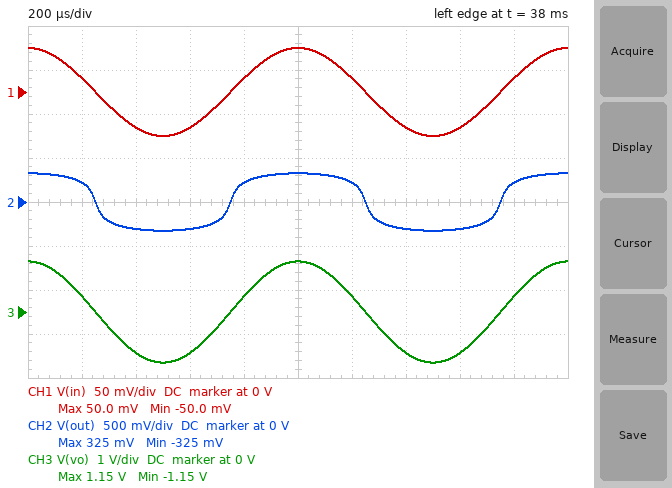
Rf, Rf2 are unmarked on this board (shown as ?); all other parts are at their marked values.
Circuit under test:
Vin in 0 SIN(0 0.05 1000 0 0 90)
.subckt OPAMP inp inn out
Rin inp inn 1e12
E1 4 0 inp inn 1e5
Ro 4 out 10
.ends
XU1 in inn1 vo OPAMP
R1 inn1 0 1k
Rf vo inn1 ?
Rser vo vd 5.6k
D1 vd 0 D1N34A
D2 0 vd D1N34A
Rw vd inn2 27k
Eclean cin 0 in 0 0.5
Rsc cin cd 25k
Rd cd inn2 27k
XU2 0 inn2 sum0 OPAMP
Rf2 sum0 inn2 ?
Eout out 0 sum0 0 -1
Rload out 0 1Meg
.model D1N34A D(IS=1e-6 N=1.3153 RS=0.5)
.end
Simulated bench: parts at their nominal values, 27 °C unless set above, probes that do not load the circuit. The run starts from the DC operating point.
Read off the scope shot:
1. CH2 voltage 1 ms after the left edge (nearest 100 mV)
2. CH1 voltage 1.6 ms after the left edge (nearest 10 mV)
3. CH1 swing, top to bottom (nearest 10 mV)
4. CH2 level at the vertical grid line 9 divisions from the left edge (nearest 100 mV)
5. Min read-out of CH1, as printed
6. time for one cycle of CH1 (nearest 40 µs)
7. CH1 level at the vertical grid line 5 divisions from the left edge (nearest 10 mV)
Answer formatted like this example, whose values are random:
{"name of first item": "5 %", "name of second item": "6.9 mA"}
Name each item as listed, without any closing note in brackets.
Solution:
{"CH2 voltage 1 ms after the left edge": "300 mV", "CH1 voltage 1.6 ms after the left edge": "-40 mV", "CH1 swing, top to bottom": "100 mV", "CH2 level at the vertical grid line 9 divisions from the left edge": "200 mV", "Min read-out of CH1, as printed": "-50.0 mV", "time for one cycle of CH1": "1.00 ms", "CH1 level at the vertical grid line 5 divisions from the left edge": "50 mV"}
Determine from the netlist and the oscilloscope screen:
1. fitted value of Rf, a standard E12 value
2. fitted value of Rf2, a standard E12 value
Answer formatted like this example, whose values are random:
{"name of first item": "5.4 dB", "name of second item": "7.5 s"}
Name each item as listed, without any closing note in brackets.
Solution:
{"fitted value of Rf, a standard E12 value": "22 kΩ", "fitted value of Rf2, a standard E12 value": "47 kΩ"}
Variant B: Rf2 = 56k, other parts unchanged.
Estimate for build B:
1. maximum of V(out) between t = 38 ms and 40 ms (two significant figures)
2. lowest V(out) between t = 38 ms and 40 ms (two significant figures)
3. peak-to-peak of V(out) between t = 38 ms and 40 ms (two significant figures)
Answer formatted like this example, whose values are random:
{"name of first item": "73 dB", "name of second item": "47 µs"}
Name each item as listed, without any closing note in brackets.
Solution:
{"maximum of V(out) between t = 38 ms and 40 ms": "390 mV", "lowest V(out) between t = 38 ms and 40 ms": "-390 mV", "peak-to-peak of V(out) between t = 38 ms and 40 ms": "780 mV"}
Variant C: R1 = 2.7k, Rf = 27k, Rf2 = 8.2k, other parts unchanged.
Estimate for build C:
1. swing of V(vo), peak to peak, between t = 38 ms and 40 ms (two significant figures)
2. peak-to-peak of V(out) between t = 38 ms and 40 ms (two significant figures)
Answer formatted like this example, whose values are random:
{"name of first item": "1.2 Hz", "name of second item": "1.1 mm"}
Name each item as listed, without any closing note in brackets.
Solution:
{"swing of V(vo), peak to peak, between t = 38 ms and 40 ms": "1.1 V", "peak-to-peak of V(out) between t = 38 ms and 40 ms": "95 mV"}
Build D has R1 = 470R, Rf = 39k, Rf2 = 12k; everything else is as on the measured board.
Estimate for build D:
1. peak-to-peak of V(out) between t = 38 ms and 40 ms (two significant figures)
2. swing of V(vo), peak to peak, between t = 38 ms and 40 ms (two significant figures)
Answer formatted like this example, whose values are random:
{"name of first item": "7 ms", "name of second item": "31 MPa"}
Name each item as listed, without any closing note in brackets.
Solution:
{"peak-to-peak of V(out) between t = 38 ms and 40 ms": "210 mV", "swing of V(vo), peak to peak, between t = 38 ms and 40 ms": "8.4 V"}
